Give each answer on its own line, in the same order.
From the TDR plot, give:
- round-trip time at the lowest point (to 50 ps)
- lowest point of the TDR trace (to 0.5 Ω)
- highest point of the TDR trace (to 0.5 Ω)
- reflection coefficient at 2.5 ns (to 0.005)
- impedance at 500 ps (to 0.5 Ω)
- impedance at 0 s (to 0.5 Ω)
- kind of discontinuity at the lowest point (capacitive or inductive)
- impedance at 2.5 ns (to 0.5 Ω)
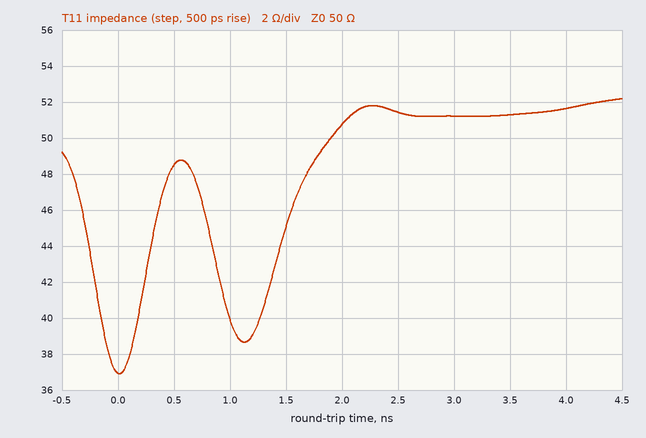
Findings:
0 ps
37.0 Ω
52.0 Ω
+0.015
48.5 Ω
37.0 Ω
capacitive
51.5 Ω
